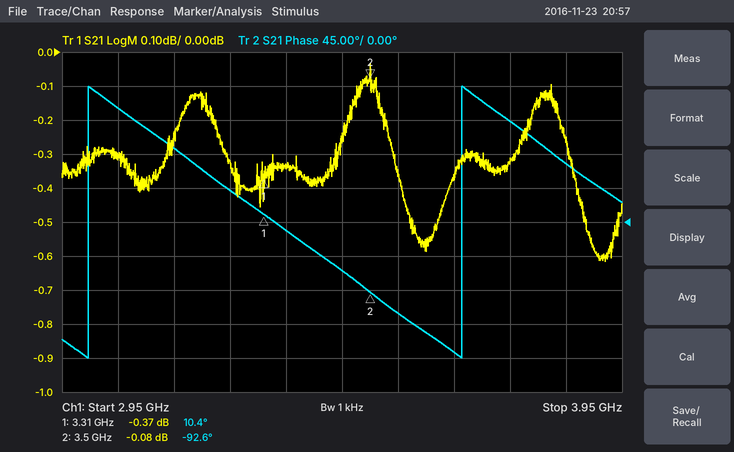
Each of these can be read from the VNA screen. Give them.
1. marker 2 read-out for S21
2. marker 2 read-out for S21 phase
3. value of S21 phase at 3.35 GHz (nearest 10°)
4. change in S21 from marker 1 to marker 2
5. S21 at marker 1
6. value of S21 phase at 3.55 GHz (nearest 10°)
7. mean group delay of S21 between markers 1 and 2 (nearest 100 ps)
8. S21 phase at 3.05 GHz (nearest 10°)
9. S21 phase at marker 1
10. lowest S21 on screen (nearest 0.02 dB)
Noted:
-0.08 dB
-92.6°
-10°
0.29 dB
-0.37 dB
-120°
1.5 ns
150°
10.4°
-0.62 dB
